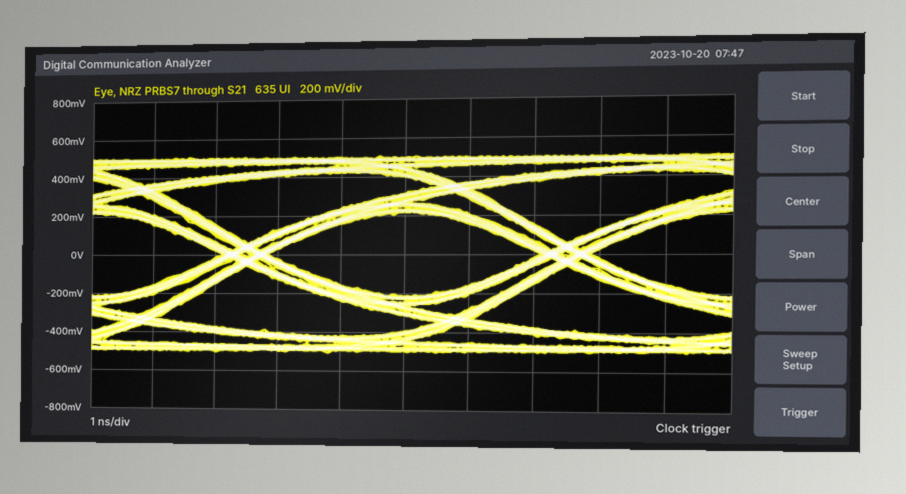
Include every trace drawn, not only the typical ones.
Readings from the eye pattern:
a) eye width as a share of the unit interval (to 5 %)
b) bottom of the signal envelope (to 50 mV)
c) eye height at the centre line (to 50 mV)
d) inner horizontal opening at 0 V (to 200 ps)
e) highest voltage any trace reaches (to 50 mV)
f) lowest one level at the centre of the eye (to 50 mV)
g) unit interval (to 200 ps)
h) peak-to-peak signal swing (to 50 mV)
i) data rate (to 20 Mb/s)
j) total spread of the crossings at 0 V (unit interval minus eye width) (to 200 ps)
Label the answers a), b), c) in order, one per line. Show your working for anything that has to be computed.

a) 4.2 ns / 5.0 ns ≈ 84.0 %, so 85 % to the nearest 5 %
b) -500 mV
c) 450 mV
d) 4.2 ns
e) 500 mV
f) 200 mV
g) 5.0 ns
h) 1.00 V
i) 200 Mb/s
j) 800 ps
